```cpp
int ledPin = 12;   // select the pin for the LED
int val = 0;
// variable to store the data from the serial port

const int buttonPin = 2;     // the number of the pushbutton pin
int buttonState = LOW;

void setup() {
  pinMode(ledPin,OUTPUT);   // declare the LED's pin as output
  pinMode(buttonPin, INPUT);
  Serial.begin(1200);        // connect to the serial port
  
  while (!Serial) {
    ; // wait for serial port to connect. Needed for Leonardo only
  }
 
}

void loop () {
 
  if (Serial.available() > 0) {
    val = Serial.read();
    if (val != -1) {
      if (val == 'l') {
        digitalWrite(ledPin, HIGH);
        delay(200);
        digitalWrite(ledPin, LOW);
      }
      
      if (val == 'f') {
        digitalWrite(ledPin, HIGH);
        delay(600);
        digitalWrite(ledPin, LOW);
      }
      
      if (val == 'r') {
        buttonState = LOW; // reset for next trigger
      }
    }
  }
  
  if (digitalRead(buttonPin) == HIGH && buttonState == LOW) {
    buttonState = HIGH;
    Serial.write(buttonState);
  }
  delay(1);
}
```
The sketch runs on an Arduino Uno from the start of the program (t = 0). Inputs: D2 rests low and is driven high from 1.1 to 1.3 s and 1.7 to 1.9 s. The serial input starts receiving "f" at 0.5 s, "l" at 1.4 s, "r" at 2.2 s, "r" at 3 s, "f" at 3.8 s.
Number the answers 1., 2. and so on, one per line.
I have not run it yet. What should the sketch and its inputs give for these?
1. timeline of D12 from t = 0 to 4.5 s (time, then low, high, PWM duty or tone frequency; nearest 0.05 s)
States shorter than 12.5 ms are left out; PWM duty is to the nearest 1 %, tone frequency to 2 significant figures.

1. 0 s low; 0.5 s high; 1.1 s low; 1.4 s high; 1.6 s low; 3.8 s high; 4.4 s low
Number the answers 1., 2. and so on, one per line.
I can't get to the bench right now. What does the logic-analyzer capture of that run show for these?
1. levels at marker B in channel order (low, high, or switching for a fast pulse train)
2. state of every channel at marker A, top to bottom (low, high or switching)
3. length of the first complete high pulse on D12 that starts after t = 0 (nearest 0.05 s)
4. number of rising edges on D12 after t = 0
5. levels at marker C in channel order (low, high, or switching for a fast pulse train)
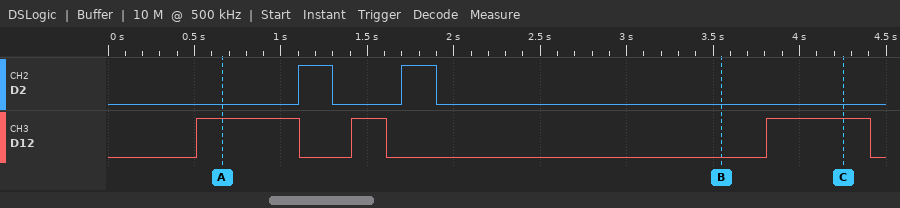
1. D2 low, D12 low
2. D2 low, D12 high
3. 0.60 s
4. 3
5. D2 low, D12 high
